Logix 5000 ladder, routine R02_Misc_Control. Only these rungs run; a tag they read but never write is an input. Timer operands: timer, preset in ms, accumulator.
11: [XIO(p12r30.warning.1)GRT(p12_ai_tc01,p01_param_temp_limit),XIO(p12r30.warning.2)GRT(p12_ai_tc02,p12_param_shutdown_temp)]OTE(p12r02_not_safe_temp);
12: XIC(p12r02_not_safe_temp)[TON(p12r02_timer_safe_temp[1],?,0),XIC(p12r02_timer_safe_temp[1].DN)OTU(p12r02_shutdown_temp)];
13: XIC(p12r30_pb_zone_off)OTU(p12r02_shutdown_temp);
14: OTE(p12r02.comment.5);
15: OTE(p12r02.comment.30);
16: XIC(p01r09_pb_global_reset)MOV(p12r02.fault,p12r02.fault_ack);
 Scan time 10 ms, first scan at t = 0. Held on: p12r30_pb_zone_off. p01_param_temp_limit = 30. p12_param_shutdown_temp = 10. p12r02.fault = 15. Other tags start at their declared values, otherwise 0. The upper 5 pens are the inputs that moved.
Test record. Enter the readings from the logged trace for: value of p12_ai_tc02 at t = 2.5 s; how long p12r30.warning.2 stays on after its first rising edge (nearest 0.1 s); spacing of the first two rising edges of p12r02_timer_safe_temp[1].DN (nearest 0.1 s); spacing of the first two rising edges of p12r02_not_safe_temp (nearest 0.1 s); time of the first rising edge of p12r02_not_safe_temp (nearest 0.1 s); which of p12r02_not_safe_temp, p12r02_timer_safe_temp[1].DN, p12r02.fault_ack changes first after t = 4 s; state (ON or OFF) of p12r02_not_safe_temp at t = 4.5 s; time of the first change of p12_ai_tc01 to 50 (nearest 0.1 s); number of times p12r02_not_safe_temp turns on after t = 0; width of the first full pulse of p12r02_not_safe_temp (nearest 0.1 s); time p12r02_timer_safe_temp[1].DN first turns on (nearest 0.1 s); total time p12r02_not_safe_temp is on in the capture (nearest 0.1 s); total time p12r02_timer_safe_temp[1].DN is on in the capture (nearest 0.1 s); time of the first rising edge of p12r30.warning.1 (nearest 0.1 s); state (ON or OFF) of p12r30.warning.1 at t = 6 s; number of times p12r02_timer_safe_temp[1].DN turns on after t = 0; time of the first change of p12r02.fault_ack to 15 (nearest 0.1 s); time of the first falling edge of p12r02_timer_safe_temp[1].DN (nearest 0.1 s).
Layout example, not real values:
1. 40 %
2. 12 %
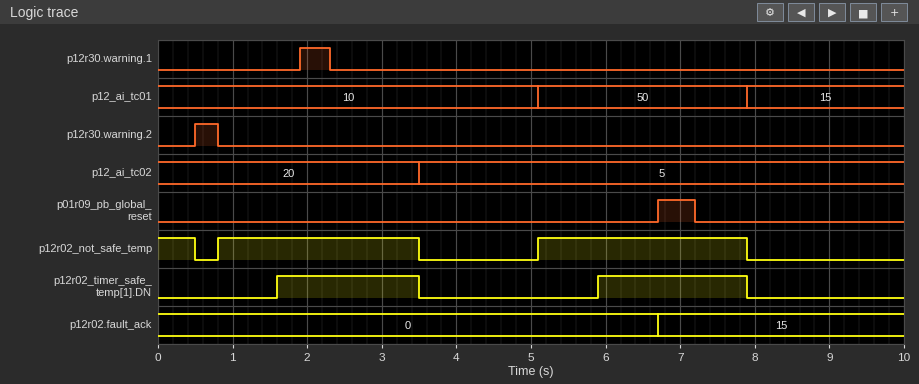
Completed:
1. 20
2. 0.3 s
3. 4.3 s
4. 4.3 s
5. 0.8 s
6. p12r02_not_safe_temp
7. OFF
8. 5.1 s
9. 2
10. 2.7 s
11. 1.6 s
12. 6.0 s
13. 3.9 s
14. 1.9 s
15. OFF
16. 2
17. 6.7 s
18. 3.5 s
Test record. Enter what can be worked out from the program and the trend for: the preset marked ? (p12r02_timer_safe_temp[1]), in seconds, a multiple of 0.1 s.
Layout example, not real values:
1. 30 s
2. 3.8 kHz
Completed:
1. 0.8 s
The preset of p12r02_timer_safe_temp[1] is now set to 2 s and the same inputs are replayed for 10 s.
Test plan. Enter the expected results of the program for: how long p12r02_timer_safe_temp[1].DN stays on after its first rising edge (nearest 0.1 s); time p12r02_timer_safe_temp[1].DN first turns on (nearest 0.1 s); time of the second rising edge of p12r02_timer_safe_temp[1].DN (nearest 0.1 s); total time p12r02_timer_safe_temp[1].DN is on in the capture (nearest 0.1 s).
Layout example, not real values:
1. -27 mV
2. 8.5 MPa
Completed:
1. 0.7 s
2. 2.8 s
3. 7.1 s
4. 1.5 s
